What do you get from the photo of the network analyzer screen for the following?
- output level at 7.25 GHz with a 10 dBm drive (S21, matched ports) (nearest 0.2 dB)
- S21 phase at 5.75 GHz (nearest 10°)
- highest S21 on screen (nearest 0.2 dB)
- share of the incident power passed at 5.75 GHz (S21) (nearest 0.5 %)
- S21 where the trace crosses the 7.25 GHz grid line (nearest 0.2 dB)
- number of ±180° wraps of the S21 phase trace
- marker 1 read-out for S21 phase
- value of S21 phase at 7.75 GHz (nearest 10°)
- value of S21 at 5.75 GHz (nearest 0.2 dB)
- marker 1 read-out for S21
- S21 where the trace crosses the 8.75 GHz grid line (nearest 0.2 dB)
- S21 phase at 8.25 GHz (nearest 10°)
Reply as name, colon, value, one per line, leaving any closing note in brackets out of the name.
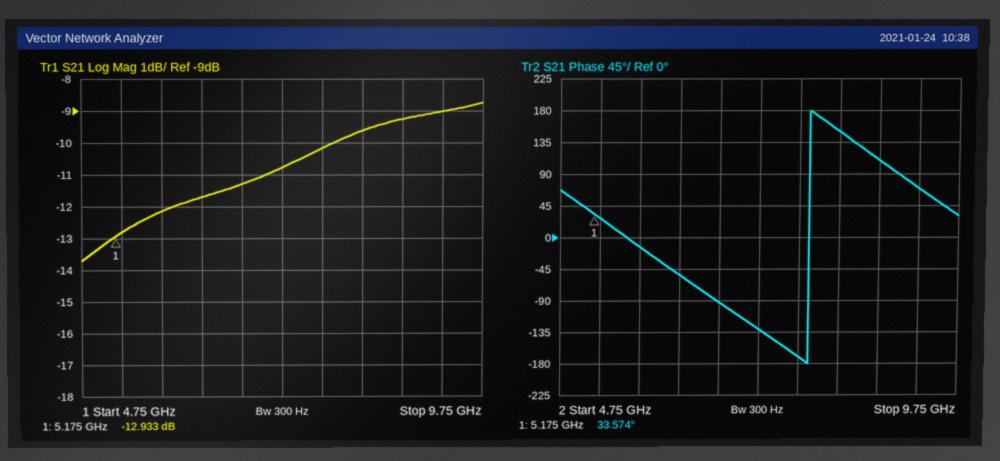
output level at 7.25 GHz with a 10 dBm drive (S21, matched ports): -0.8 dBm
S21 phase at 5.75 GHz: -10°
highest S21 on screen: -8.8 dB
share of the incident power passed at 5.75 GHz (S21): 6.0 %
S21 where the trace crosses the 7.25 GHz grid line: -10.8 dB
number of ±180° wraps of the S21 phase trace: 1
marker 1 read-out for S21 phase: 33.574°
value of S21 phase at 7.75 GHz: -170°
value of S21 at 5.75 GHz: -12.2 dB
marker 1 read-out for S21: -12.933 dB
S21 where the trace crosses the 8.75 GHz grid line: -9.2 dB
S21 phase at 8.25 GHz: 150°
